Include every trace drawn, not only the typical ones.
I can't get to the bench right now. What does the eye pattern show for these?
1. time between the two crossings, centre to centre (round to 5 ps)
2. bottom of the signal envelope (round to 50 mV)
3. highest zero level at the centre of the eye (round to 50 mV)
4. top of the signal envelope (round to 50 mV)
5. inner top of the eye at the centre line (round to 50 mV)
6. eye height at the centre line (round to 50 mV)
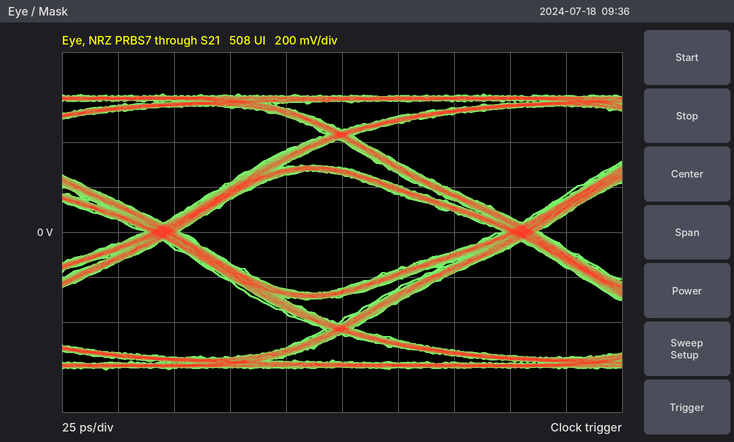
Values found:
160 ps
-600 mV
-250 mV
600 mV
250 mV
500 mV
